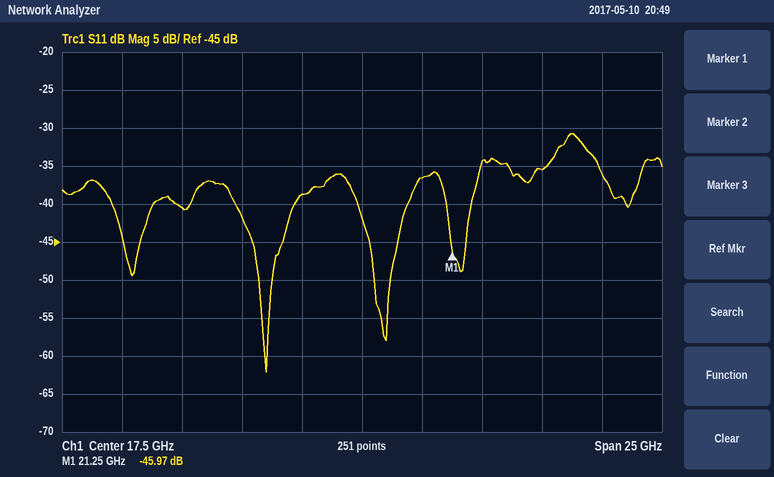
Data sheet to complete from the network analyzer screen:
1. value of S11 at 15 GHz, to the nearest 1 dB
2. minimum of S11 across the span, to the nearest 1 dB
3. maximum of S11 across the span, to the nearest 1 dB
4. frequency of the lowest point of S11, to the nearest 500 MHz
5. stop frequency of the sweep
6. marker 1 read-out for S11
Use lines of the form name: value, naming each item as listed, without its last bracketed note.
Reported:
value of S11 at 15 GHz, to the nearest 1 dB: -39 dB
minimum of S11 across the span, to the nearest 1 dB: -62 dB
maximum of S11 across the span, to the nearest 1 dB: -31 dB
frequency of the lowest point of S11, to the nearest 500 MHz: 13.5 GHz
stop frequency of the sweep: 30 GHz
marker 1 read-out for S11: -45.97 dB
